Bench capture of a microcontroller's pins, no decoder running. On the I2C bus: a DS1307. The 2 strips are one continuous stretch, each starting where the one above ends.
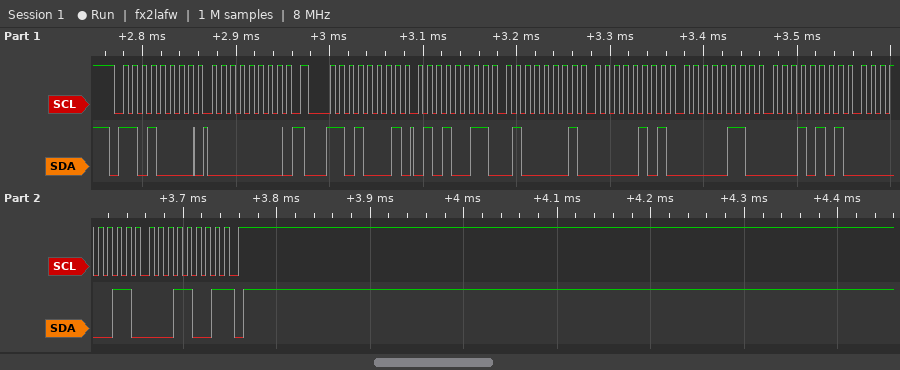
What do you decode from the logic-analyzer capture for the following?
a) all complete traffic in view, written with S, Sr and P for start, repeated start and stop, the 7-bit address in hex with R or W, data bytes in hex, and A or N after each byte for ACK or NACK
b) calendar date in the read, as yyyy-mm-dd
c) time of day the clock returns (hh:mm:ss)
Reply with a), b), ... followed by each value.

a) S 68W A 00 A Sr 68R A 53 A 41 A 05 A 06 A 15 A 03 A 19 N P
b) 2019-03-15
c) 05:41:53
